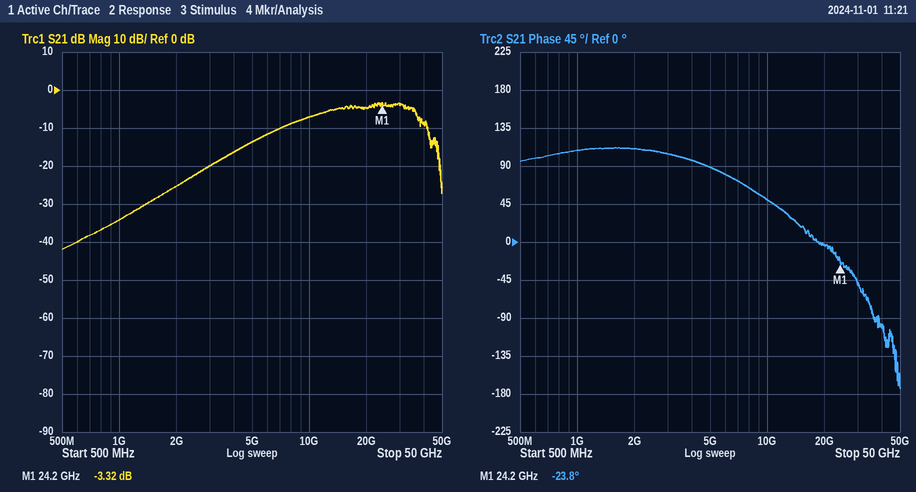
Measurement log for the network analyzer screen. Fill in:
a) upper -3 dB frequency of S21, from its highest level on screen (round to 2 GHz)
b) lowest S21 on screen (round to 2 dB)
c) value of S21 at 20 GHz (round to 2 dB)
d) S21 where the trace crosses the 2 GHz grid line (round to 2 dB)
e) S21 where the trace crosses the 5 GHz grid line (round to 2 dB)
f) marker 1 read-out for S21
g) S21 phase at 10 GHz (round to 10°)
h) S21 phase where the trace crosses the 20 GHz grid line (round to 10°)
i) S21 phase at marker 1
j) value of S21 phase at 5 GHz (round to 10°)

36 GHz
-42 dB
-4 dB
-26 dB
-14 dB
-3.32 dB
50°
0°
-23.8°
90°
